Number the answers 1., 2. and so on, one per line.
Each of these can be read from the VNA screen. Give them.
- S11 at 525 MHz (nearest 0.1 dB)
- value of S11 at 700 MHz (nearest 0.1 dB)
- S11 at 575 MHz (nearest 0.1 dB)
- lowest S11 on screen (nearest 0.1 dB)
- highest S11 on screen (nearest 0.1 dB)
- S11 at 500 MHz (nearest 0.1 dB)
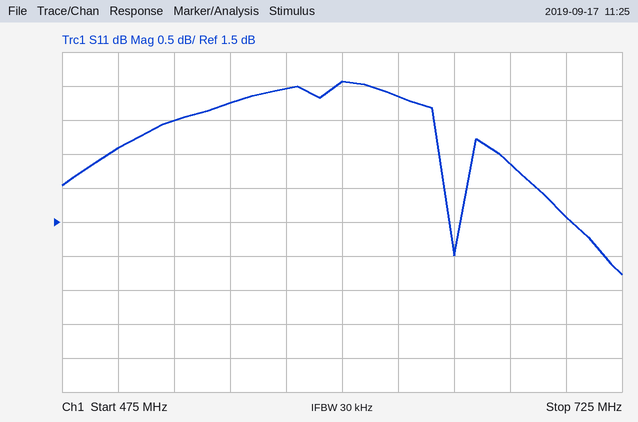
1. 3.0 dB
2. 1.6 dB
3. 3.5 dB
4. 0.7 dB
5. 3.6 dB
6. 2.6 dB
